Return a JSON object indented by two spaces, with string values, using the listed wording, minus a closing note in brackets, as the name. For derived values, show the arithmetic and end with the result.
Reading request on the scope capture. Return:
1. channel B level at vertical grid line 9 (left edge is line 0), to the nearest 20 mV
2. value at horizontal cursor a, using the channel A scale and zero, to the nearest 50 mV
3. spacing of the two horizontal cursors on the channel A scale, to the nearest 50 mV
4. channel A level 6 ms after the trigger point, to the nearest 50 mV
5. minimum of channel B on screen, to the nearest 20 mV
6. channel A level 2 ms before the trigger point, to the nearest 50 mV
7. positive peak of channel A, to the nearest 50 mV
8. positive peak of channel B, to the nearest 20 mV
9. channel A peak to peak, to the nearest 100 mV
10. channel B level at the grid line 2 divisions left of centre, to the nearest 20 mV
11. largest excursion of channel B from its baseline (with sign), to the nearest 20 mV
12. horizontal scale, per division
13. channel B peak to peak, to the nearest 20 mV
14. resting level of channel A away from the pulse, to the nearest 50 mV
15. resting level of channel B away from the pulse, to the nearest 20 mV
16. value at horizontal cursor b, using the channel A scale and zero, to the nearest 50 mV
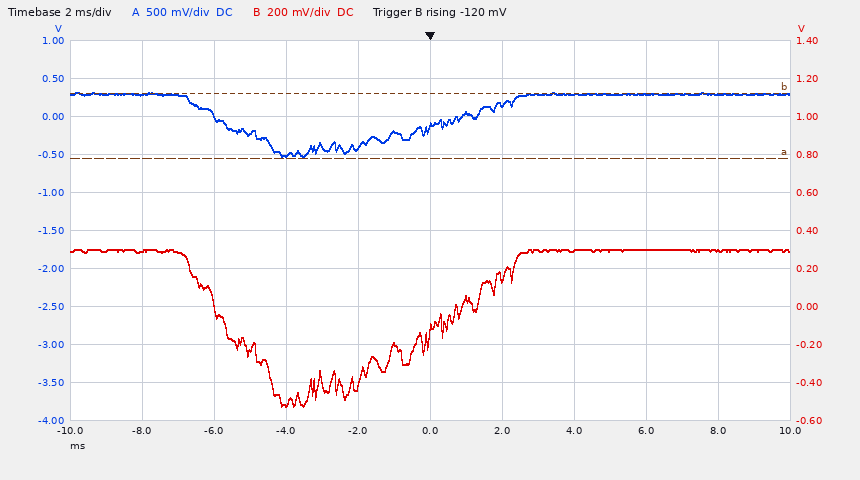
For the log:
{
  "channel B level at vertical grid line 9 (left edge is line 0), to the nearest 20 mV": "300 mV",
  "value at horizontal cursor a, using the channel A scale and zero, to the nearest 50 mV": "-550 mV",
  "spacing of the two horizontal cursors on the channel A scale, to the nearest 50 mV": "850 mV",
  "channel A level 6 ms after the trigger point, to the nearest 50 mV": "300 mV",
  "minimum of channel B on screen, to the nearest 20 mV": "-520 mV",
  "channel A level 2 ms before the trigger point, to the nearest 50 mV": "-400 mV",
  "positive peak of channel A, to the nearest 50 mV": "300 mV",
  "positive peak of channel B, to the nearest 20 mV": "300 mV",
  "channel A peak to peak, to the nearest 100 mV": "800 mV",
  "channel B level at the grid line 2 divisions left of centre, to the nearest 20 mV": "-500 mV",
  "largest excursion of channel B from its baseline (with sign), to the nearest 20 mV": "-520 mV − (300 mV) = -820 mV",
  "horizontal scale, per division": "2 ms",
  "channel B peak to peak, to the nearest 20 mV": "300 mV − (-520 mV) = 820 mV",
  "resting level of channel A away from the pulse, to the nearest 50 mV": "300 mV",
  "resting level of channel B away from the pulse, to the nearest 20 mV": "300 mV",
  "value at horizontal cursor b, using the channel A scale and zero, to the nearest 50 mV": "300 mV"
}
